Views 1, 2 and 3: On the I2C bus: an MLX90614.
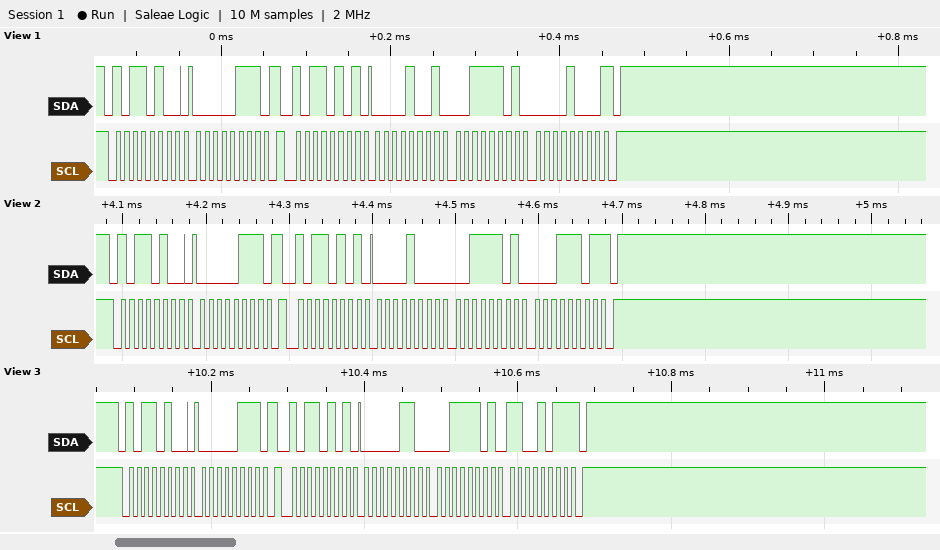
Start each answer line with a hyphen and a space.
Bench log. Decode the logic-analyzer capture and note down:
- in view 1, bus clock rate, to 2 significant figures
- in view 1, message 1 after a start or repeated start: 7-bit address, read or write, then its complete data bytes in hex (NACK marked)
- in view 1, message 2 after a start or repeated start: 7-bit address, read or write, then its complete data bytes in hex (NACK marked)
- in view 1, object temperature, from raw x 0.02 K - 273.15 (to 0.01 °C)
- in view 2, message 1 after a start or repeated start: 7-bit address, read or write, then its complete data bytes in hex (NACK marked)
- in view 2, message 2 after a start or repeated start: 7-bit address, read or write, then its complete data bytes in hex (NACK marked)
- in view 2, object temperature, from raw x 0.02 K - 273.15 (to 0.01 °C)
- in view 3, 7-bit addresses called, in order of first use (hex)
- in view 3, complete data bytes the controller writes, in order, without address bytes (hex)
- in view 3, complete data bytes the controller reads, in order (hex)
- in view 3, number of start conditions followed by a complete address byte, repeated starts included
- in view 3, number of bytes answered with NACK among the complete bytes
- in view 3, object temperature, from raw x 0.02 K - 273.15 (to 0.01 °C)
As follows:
- 100 kHz
- 0x5A write: 07
- 0x5A read: 09 3D 08 NACK
- 39.35 °C
- 0x5A write: 07
- 0x5A read: 08 3D 1D NACK
- 39.33 °C
- 0x5A
- 07
- 06 3D CB
- 2
- 1
- 39.29 °C
